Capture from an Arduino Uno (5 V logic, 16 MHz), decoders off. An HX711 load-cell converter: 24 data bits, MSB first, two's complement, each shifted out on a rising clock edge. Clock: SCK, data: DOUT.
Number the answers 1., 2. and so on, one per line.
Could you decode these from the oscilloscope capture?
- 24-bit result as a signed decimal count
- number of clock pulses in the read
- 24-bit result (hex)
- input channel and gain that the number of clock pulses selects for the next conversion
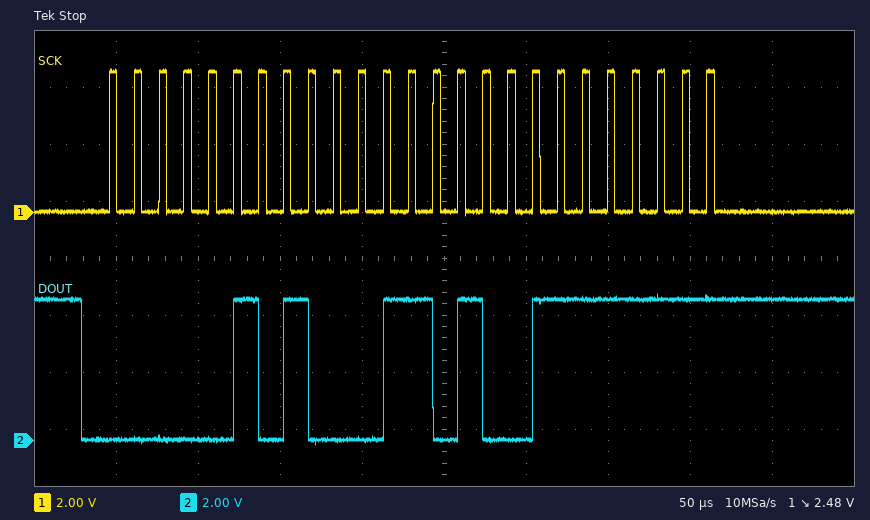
1. 334463
2. 25
3. 0x051A7F
4. channel A, gain 128
